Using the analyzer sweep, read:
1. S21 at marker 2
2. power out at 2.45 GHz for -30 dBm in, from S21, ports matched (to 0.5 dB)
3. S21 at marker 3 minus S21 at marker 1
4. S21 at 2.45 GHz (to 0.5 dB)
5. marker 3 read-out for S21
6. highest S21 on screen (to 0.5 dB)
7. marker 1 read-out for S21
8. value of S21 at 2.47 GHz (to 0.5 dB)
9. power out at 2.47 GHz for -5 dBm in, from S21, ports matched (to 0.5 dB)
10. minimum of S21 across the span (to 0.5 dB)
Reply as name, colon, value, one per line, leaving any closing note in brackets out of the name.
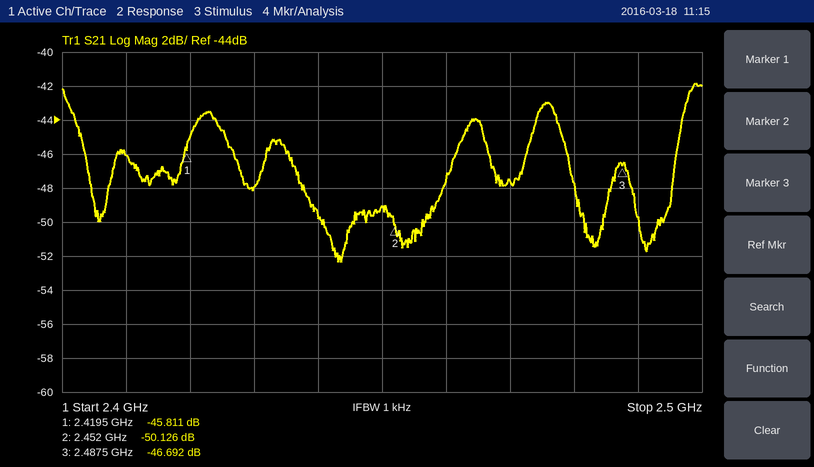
S21 at marker 2: -50.126 dB
power out at 2.45 GHz for -30 dBm in, from S21, ports matched: -79.0 dBm
S21 at marker 3 minus S21 at marker 1: -0.881 dB
S21 at 2.45 GHz: -49.0 dB
marker 3 read-out for S21: -46.692 dB
highest S21 on screen: -42.0 dB
marker 1 read-out for S21: -45.811 dB
value of S21 at 2.47 GHz: -47.5 dB
power out at 2.47 GHz for -5 dBm in, from S21, ports matched: -52.5 dBm
minimum of S21 across the span: -52.5 dB
